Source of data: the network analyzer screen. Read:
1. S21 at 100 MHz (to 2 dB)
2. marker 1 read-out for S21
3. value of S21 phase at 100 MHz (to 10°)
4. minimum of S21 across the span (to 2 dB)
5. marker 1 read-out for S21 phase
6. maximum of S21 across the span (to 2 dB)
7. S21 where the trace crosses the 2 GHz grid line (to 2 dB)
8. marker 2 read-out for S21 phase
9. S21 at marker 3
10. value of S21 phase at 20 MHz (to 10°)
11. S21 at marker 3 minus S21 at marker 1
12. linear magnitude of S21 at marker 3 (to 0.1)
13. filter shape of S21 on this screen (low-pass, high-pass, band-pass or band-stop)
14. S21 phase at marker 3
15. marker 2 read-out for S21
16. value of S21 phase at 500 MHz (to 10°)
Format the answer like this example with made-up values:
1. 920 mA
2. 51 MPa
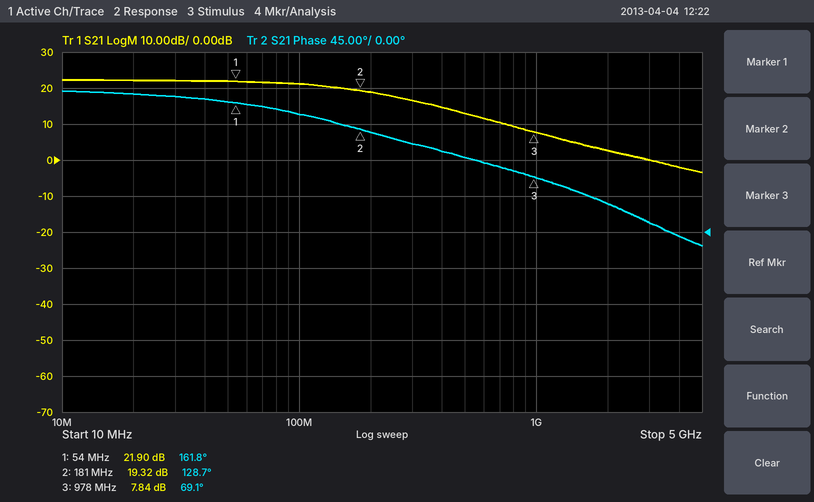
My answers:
1. 22 dB
2. 21.90 dB
3. 150°
4. -4 dB
5. 161.8°
6. 22 dB
7. 2 dB
8. 128.7°
9. 7.84 dB
10. 170°
11. -14.06 dB
12. 2.5
13. low-pass
14. 69.1°
15. 19.32 dB
16. 90°
